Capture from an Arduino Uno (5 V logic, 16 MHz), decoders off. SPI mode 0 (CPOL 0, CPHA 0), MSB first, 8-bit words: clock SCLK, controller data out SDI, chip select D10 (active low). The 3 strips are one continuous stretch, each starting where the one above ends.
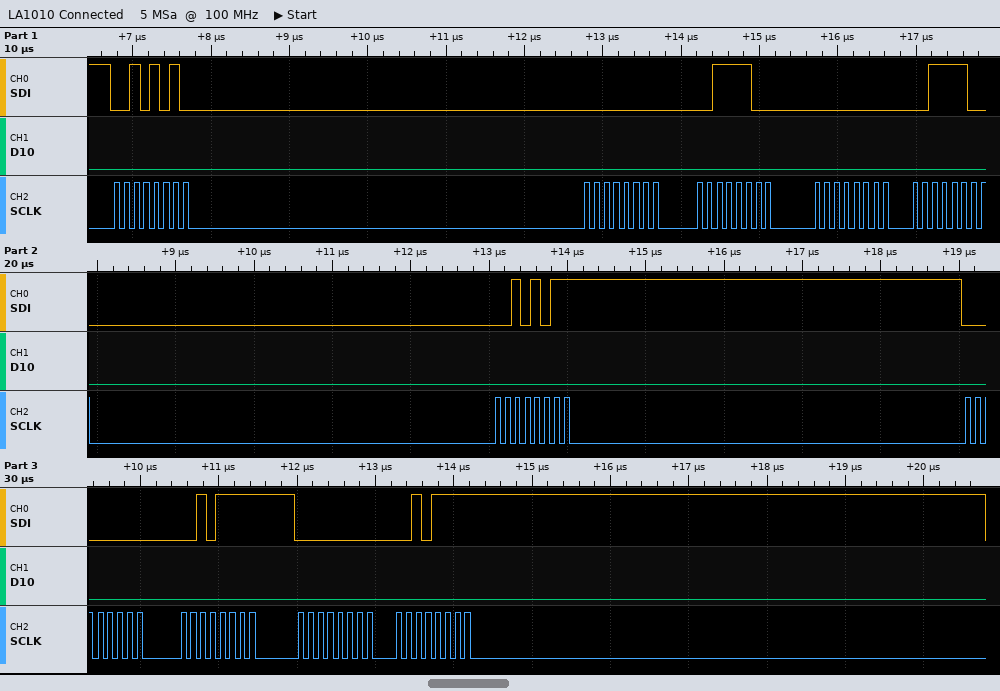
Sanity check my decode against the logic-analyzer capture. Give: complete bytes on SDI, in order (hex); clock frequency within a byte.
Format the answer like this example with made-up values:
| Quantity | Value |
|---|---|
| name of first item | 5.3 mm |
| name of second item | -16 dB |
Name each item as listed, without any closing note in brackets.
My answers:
| Quantity | Value |
|---|---|
| complete bytes on SDI, in order | 2A 00 3C 00 3C 2B 00 2F 00 2F |
| clock frequency within a byte | 8 MHz |
